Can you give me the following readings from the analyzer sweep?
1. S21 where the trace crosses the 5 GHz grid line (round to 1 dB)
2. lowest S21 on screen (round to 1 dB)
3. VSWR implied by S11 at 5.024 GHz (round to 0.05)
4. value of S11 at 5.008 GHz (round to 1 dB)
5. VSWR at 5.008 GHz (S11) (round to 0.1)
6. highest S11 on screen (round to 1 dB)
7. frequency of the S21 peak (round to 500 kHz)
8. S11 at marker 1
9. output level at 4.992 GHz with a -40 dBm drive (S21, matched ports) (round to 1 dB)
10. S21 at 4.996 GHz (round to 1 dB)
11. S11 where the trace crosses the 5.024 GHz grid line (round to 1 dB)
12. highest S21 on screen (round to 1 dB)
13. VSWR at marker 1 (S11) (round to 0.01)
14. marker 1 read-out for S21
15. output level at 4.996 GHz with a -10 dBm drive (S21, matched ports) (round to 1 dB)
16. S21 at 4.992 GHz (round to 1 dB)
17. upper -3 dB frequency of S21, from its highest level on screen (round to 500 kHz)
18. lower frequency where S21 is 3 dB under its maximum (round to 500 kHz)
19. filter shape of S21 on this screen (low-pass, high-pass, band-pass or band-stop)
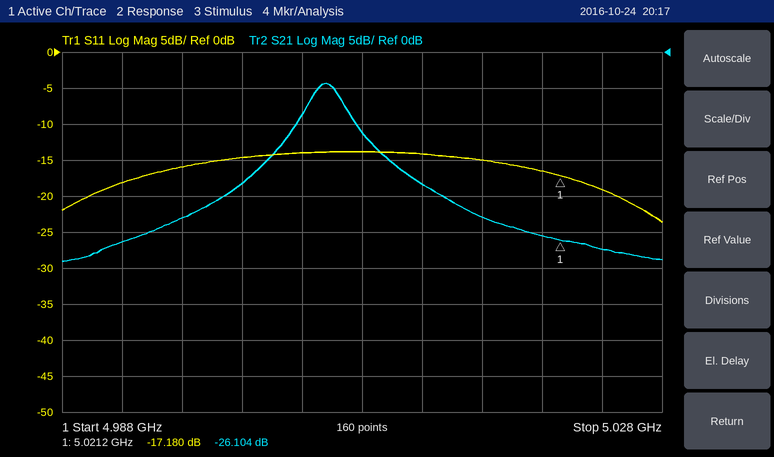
-18 dB
-29 dB
1.25
-14 dB
1.5
-14 dB
5.0055 GHz
-17.180 dB
-66 dBm
-23 dB
-19 dB
-4 dB
1.32
-26.104 dB
-33 dBm
-26 dB
5.0070 GHz
5.0045 GHz
band-pass
